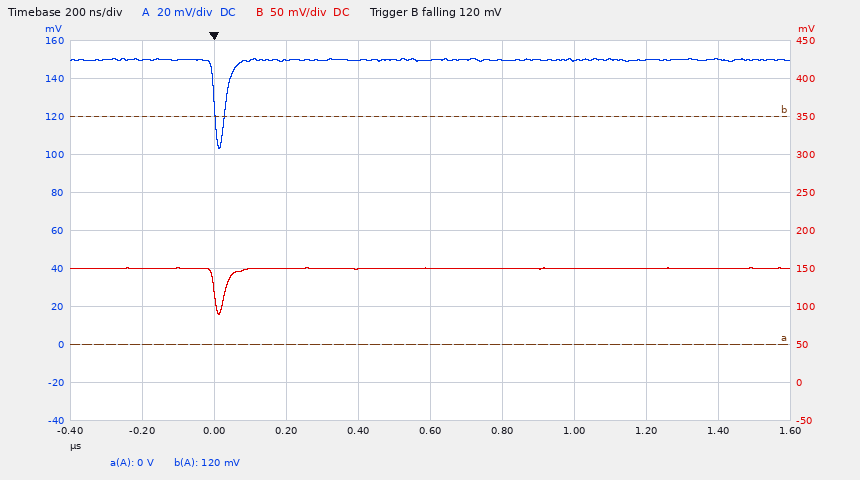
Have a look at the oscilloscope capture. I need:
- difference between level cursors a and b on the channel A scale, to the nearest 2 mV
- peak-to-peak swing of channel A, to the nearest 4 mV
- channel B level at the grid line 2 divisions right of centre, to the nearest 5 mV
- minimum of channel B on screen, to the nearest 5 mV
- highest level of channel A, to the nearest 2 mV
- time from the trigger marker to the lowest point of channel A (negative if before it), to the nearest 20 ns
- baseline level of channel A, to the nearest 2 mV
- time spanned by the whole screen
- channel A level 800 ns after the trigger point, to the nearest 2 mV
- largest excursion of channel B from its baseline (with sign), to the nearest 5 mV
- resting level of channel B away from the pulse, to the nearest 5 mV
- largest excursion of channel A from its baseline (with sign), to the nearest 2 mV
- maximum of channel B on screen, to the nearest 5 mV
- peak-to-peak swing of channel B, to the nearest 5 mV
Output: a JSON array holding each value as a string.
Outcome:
["120 mV", "48 mV", "150 mV", "90 mV", "150 mV", "+20 ns", "150 mV", "2 µs", "150 mV", "-60 mV", "150 mV", "-46 mV", "150 mV", "60 mV"]
